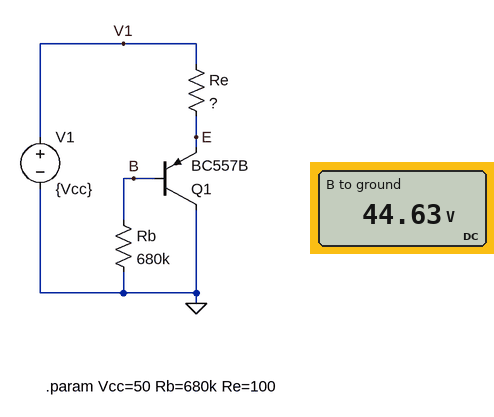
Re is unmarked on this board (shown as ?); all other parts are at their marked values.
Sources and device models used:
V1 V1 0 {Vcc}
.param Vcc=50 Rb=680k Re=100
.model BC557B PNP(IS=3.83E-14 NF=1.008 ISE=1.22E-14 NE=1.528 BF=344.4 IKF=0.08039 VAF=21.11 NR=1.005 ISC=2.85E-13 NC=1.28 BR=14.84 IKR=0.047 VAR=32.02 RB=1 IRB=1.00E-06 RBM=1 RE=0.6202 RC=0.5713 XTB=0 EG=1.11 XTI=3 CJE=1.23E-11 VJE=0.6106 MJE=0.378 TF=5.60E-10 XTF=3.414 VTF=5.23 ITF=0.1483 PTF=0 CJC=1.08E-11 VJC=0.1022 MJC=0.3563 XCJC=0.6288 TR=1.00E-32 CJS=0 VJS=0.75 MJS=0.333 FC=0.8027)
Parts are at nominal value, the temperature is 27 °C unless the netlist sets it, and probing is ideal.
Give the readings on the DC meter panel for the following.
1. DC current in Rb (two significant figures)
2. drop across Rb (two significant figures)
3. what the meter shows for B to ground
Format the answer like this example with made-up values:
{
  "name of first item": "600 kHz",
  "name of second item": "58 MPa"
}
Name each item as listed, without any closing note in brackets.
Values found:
{
  "DC current in Rb": "66 µA",
  "drop across Rb": "45 V",
  "what the meter shows for B to ground": "44.63 V"
}
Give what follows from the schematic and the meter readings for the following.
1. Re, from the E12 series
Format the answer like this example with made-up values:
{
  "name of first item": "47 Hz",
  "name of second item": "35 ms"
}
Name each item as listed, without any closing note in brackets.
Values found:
{
  "Re, from the E12 series": "82 Ω"
}
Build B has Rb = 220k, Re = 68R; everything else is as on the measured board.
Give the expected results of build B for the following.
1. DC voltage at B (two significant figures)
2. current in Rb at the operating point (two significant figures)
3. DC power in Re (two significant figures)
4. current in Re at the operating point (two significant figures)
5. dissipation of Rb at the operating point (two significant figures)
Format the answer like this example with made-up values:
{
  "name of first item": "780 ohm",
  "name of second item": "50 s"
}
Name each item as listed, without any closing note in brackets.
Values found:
{
  "DC voltage at B": "41 V",
  "current in Rb at the operating point": "190 µA",
  "DC power in Re": "1.0 W",
  "current in Re at the operating point": "120 mA",
  "dissipation of Rb at the operating point": "7.6 mW"
}
